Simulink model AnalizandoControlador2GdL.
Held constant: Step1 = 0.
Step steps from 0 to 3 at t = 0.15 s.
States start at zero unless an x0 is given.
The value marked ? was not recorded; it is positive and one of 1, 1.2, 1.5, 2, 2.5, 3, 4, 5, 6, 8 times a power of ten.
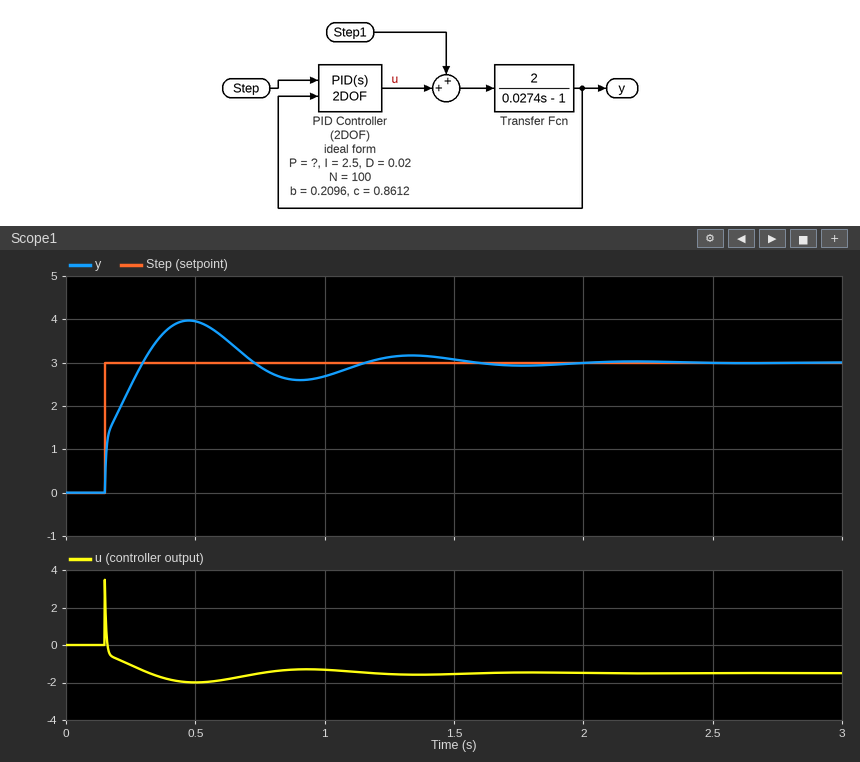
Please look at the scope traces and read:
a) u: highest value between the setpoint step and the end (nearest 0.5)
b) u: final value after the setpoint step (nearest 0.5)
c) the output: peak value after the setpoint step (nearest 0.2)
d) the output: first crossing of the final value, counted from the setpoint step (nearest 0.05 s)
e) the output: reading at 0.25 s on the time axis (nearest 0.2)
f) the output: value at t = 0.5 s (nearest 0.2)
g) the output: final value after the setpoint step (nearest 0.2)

3.5
-1.5
4.0
0.15 s
2.4
4.0
3.0
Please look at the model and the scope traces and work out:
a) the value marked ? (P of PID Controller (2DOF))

0.6
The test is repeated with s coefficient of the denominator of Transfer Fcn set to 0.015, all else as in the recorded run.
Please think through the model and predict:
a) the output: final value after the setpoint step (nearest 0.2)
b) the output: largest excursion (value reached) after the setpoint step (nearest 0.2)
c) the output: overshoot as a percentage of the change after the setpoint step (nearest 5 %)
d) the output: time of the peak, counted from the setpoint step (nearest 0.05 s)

3.0
3.8
25 %
0.25 s
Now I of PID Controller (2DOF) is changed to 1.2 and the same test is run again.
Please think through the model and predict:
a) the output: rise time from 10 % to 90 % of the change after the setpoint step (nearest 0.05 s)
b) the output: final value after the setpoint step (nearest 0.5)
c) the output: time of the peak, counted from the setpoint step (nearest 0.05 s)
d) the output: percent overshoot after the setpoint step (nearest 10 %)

0.15 s
3.0
0.45 s
30 %
